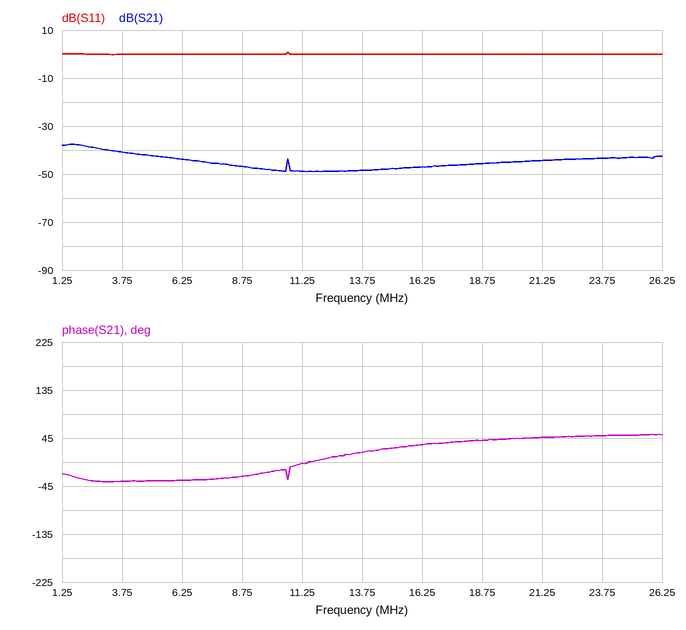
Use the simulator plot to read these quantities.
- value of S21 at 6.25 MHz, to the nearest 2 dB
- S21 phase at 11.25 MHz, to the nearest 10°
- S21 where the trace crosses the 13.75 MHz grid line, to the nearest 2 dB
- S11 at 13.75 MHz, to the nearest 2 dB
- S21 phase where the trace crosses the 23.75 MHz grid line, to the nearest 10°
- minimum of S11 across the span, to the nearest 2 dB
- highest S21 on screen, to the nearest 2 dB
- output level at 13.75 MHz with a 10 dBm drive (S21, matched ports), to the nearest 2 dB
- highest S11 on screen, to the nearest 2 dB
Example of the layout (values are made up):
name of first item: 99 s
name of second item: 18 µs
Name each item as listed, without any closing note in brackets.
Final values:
value of S21 at 6.25 MHz, to the nearest 2 dB: -44 dB
S21 phase at 11.25 MHz, to the nearest 10°: 0°
S21 where the trace crosses the 13.75 MHz grid line, to the nearest 2 dB: -48 dB
S11 at 13.75 MHz, to the nearest 2 dB: 0 dB
S21 phase where the trace crosses the 23.75 MHz grid line, to the nearest 10°: 50°
minimum of S11 across the span, to the nearest 2 dB: 0 dB
highest S21 on screen, to the nearest 2 dB: -38 dB
output level at 13.75 MHz with a 10 dBm drive (S21, matched ports), to the nearest 2 dB: -38 dBm
highest S11 on screen, to the nearest 2 dB: 0 dB
